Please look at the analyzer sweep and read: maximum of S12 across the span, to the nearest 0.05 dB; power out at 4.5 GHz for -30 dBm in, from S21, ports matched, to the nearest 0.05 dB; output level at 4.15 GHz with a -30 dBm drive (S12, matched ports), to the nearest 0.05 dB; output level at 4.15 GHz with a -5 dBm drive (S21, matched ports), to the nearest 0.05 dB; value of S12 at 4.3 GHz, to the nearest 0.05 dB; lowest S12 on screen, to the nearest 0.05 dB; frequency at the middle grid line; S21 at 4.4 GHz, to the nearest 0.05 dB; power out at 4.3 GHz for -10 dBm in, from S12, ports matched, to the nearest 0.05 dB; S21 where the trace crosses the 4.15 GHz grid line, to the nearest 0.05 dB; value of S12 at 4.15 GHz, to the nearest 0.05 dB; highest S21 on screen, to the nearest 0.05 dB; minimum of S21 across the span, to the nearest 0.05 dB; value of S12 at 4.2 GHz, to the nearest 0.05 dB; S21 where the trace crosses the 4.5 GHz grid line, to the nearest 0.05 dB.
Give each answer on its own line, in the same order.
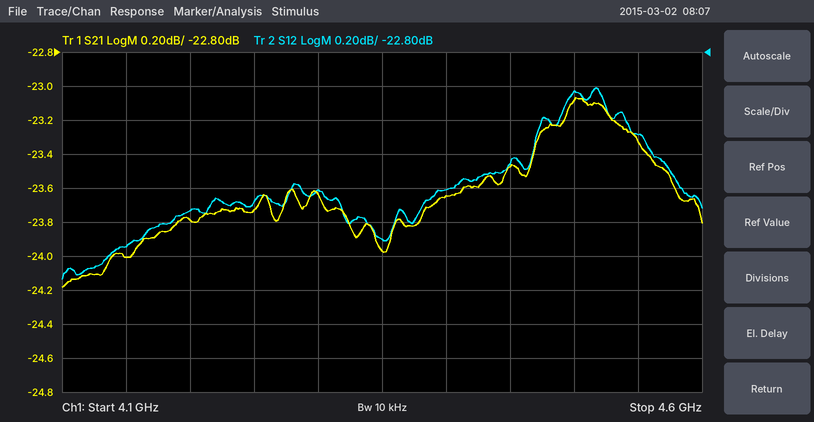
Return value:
-23.00 dB
-53.10 dBm
-53.95 dBm
-29.00 dBm
-23.60 dB
-24.15 dB
4.35 GHz
-23.65 dB
-33.60 dBm
-24.00 dB
-23.95 dB
-23.05 dB
-24.20 dB
-23.75 dB
-23.10 dB
